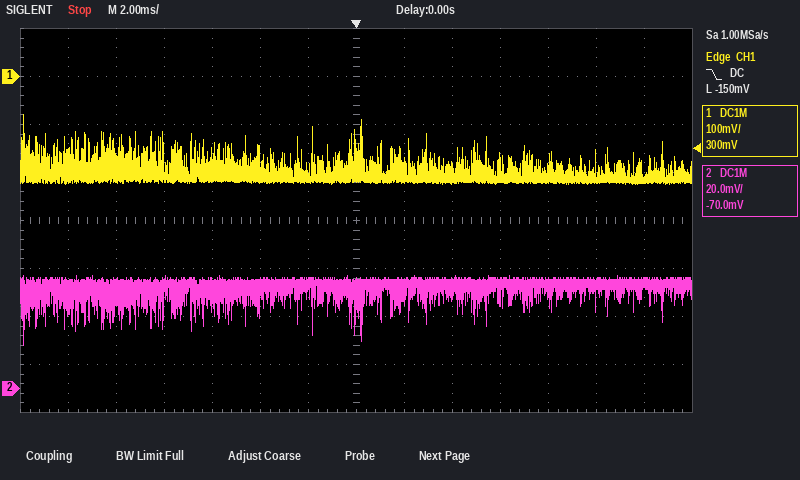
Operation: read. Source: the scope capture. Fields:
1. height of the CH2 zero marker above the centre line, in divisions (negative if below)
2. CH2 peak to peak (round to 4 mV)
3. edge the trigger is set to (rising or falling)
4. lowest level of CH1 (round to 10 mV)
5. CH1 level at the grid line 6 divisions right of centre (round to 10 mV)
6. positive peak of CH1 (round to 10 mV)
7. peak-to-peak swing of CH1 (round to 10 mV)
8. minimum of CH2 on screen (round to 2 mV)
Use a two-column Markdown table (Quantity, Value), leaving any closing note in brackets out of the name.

| Quantity | Value |
|---|---|
| height of the CH2 zero marker above the centre line, in divisions | -3.5 div |
| CH2 peak to peak | 28 mV |
| edge the trigger is set to | falling |
| lowest level of CH1 | -220 mV |
| CH1 level at the grid line 6 divisions right of centre | -210 mV |
| positive peak of CH1 | -80 mV |
| peak-to-peak swing of CH1 | 140 mV |
| minimum of CH2 on screen | 18 mV |
